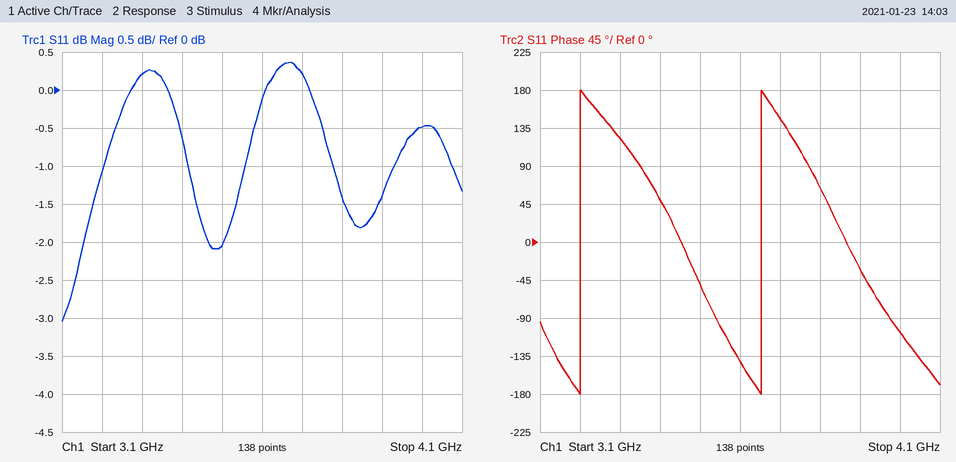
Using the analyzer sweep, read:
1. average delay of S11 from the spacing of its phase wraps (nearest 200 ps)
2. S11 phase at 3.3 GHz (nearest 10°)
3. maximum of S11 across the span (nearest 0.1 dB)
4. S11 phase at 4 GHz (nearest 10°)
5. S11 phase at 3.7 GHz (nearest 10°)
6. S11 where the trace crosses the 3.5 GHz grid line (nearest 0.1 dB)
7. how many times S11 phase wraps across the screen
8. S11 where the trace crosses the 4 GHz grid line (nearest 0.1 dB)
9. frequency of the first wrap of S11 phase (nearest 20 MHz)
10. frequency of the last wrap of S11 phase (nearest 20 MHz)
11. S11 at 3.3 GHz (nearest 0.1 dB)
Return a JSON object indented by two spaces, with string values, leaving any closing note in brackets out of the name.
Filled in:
{
  "average delay of S11 from the spacing of its phase wraps": "2.2 ns",
  "S11 phase at 3.3 GHz": "120°",
  "maximum of S11 across the span": "0.4 dB",
  "S11 phase at 4 GHz": "-110°",
  "S11 phase at 3.7 GHz": "150°",
  "S11 where the trace crosses the 3.5 GHz grid line": "-2.0 dB",
  "how many times S11 phase wraps across the screen": "2",
  "S11 where the trace crosses the 4 GHz grid line": "-0.5 dB",
  "frequency of the first wrap of S11 phase": "3.20 GHz",
  "frequency of the last wrap of S11 phase": "3.66 GHz",
  "S11 at 3.3 GHz": "0.2 dB"
}
